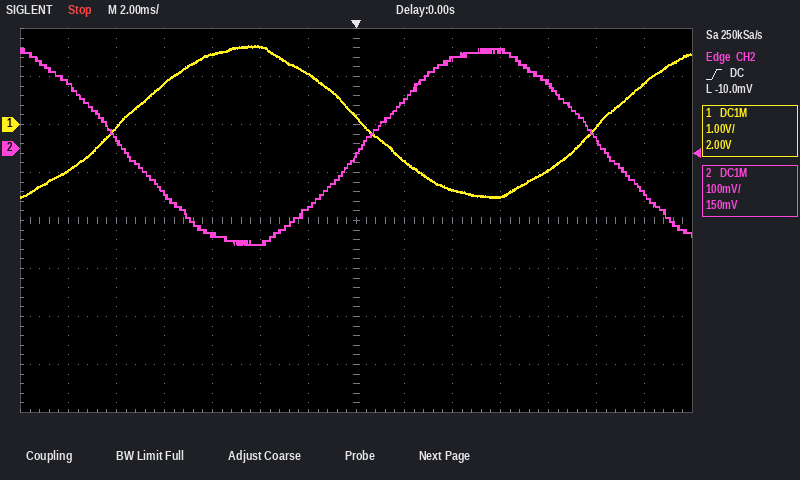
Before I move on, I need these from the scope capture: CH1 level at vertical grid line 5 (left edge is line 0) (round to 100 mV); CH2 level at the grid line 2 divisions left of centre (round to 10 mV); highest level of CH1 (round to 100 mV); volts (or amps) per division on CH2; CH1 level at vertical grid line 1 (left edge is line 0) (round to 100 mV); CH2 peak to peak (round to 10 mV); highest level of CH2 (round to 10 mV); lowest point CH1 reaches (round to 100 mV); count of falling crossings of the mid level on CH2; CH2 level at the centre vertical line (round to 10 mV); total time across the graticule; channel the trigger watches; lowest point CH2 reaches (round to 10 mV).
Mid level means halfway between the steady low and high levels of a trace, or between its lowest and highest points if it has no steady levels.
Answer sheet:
1.6 V
-200 mV
1.6 V
100 mV
-1.0 V
410 mV
210 mV
-1.5 V
2
-20 mV
28 ms
CH2
-200 mV
